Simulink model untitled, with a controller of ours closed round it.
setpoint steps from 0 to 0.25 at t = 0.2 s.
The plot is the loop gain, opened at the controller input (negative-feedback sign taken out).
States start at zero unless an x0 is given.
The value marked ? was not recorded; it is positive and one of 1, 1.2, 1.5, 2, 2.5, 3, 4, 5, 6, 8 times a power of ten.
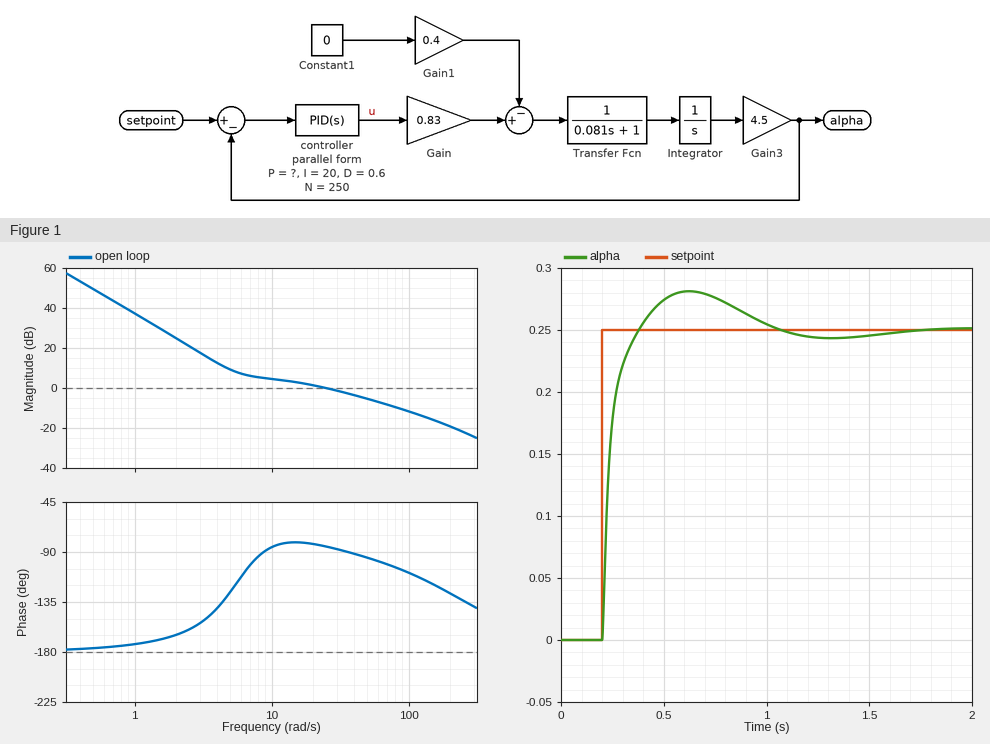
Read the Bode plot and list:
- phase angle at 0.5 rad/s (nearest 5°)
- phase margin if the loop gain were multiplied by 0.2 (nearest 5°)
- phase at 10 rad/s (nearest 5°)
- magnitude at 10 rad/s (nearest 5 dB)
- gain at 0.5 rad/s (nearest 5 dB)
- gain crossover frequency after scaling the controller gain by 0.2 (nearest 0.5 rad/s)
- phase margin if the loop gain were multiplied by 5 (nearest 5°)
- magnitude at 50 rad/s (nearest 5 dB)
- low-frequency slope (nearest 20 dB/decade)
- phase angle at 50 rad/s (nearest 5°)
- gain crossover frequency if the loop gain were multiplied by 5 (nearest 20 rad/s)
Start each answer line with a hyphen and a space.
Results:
- -175°
- 35°
- -85°
- 5 dB
- 50 dB
- 3.5 rad/s
- 65°
- -5 dB
- -40 dB/decade
- -95°
- 120 rad/s
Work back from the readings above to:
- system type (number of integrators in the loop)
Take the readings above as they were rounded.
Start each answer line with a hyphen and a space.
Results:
- 2
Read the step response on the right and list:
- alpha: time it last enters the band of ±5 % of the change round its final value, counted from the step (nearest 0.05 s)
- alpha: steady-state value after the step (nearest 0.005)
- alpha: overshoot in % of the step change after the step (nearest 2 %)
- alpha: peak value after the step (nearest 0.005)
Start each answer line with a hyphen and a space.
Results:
- 0.70 s
- 0.250
- 12 %
- 0.280
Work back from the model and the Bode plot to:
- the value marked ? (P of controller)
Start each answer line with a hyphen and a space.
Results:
- 4
